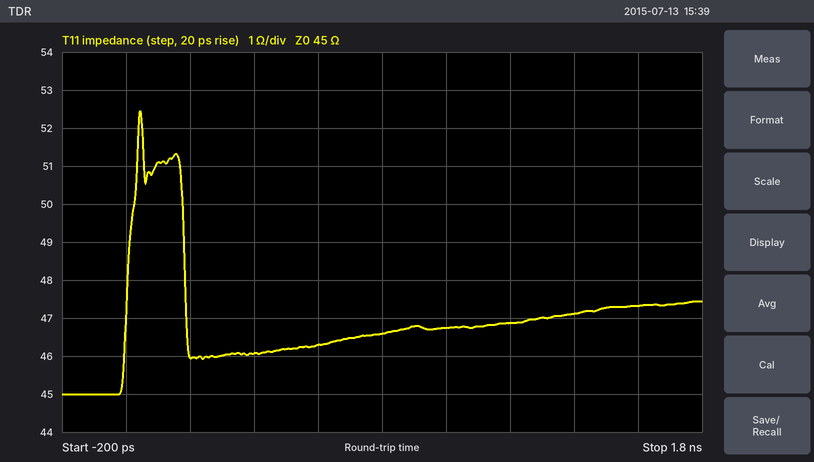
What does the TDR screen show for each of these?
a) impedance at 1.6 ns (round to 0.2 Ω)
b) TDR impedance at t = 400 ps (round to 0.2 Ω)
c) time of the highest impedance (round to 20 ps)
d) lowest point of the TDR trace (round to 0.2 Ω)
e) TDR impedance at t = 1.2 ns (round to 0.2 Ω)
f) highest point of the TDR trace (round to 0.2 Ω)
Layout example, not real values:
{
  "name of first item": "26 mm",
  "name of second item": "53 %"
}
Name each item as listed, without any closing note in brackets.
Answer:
{
  "impedance at 1.6 ns": "47.4 Ω",
  "TDR impedance at t = 400 ps": "46.0 Ω",
  "time of the highest impedance": "40 ps",
  "lowest point of the TDR trace": "45.0 Ω",
  "TDR impedance at t = 1.2 ns": "46.8 Ω",
  "highest point of the TDR trace": "52.4 Ω"
}
